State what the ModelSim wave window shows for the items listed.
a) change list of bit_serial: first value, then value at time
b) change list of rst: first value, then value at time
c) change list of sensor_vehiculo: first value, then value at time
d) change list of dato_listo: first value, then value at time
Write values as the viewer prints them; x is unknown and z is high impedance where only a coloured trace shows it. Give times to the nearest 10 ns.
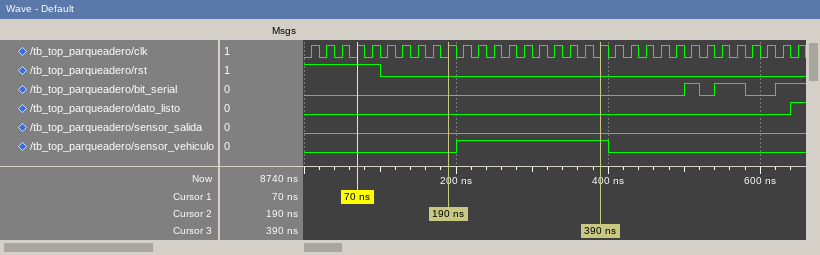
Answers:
0, 1 at 500 ns, 0 at 520 ns, 1 at 540 ns, 0 at 580 ns, 1 at 620 ns
1, 0 at 100 ns
0, 1 at 200 ns, 0 at 400 ns
0, 1 at 640 ns
